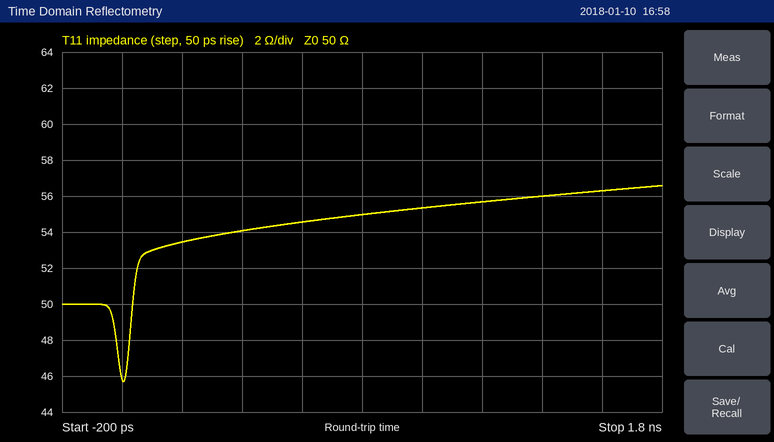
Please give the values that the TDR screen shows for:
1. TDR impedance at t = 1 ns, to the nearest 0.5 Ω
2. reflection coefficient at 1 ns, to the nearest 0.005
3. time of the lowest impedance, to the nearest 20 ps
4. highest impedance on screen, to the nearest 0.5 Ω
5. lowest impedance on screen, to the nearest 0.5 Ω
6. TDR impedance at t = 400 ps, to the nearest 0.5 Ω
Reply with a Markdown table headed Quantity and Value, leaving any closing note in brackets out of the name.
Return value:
| Quantity | Value |
|---|---|
| TDR impedance at t = 1 ns, to the nearest 0.5 Ω | 55.5 Ω |
| reflection coefficient at 1 ns, to the nearest 0.005 | +0.050 |
| time of the lowest impedance, to the nearest 20 ps | 0 ps |
| highest impedance on screen, to the nearest 0.5 Ω | 56.5 Ω |
| lowest impedance on screen, to the nearest 0.5 Ω | 45.5 Ω |
| TDR impedance at t = 400 ps, to the nearest 0.5 Ω | 54.0 Ω |
